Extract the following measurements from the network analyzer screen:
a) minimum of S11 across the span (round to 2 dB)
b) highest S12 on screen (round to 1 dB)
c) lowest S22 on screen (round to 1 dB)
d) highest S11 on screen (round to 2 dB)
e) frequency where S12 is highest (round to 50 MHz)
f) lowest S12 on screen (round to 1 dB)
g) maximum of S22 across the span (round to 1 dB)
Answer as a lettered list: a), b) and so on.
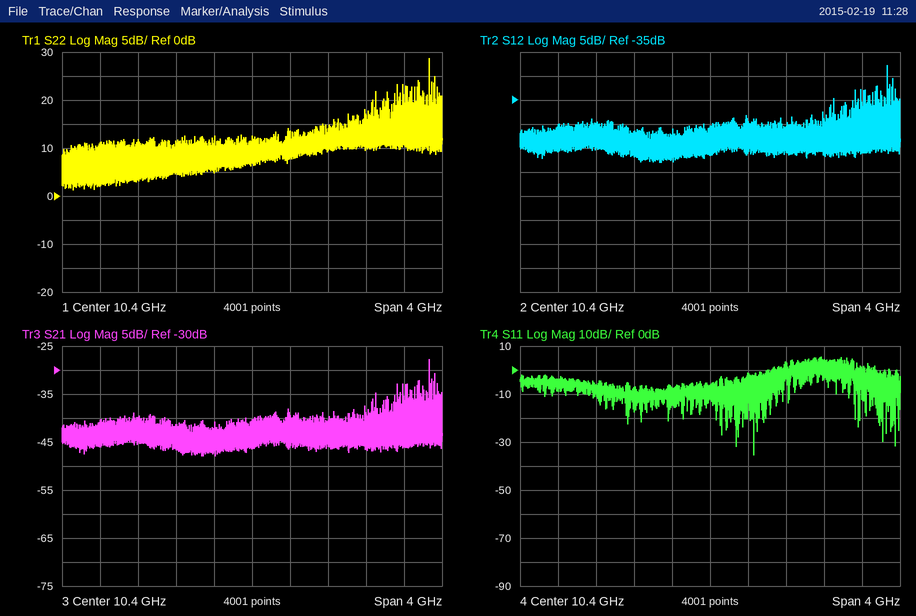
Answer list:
a) -36 dB
b) -28 dB
c) 1 dB
d) 6 dB
e) 12.25 GHz
f) -48 dB
g) 29 dB
